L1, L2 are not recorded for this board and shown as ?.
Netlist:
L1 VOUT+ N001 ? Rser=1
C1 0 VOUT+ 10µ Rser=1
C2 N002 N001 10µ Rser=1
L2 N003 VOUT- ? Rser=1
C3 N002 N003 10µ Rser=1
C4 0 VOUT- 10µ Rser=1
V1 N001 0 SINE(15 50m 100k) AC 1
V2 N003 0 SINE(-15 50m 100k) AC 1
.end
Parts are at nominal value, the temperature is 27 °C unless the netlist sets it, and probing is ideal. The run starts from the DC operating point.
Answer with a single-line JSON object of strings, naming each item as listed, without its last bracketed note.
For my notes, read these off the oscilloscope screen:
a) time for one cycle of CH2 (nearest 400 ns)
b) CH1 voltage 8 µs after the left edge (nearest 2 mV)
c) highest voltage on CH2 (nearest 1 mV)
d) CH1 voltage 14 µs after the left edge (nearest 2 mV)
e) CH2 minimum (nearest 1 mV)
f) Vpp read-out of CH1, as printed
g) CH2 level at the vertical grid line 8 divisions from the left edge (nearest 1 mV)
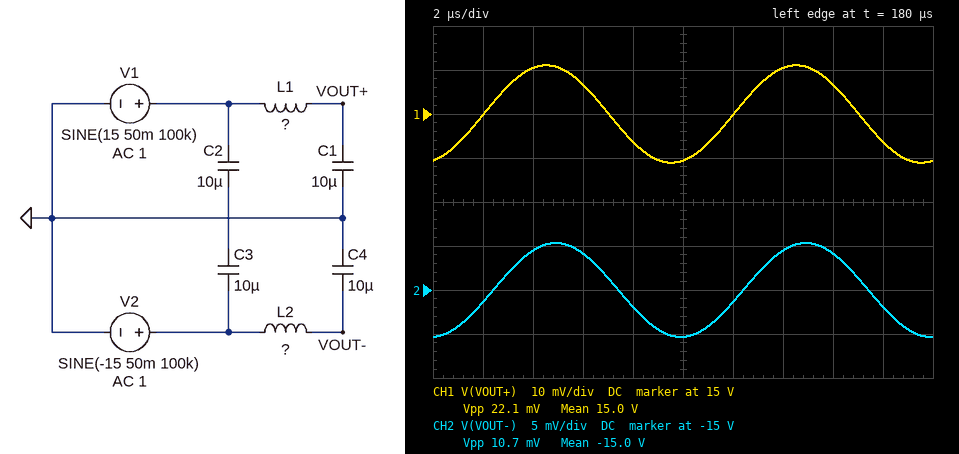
{"time for one cycle of CH2": "10.0 µs", "CH1 voltage 8 µs after the left edge": "14.994 V", "highest voltage on CH2": "-14.995 V", "CH1 voltage 14 µs after the left edge": "15.010 V", "CH2 minimum": "-15.005 V", "Vpp read-out of CH1, as printed": "22.1 mV", "CH2 level at the vertical grid line 8 divisions from the left edge": "-14.996 V"}
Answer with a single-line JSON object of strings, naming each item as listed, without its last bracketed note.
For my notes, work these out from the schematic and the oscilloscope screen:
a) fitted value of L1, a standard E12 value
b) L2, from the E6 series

{"fitted value of L1, a standard E12 value": "6.8 µH", "L2, from the E6 series": "15 µH"}
